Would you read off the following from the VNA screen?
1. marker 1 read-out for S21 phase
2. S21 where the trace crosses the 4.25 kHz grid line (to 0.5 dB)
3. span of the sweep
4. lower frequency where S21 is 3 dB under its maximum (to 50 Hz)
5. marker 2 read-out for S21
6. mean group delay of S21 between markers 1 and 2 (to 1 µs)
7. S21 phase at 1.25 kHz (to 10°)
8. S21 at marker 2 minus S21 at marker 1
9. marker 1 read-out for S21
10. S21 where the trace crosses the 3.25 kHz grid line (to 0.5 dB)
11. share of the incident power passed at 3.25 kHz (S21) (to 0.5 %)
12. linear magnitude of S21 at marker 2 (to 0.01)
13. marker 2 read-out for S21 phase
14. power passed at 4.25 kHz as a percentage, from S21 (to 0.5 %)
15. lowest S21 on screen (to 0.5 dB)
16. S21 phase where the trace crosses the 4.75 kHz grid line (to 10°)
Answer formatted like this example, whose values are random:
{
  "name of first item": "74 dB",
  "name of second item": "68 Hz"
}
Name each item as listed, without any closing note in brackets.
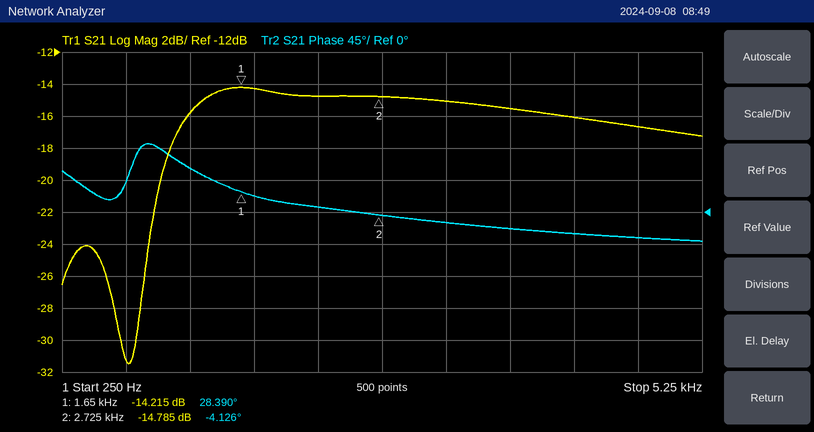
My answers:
{
  "marker 1 read-out for S21 phase": "28.390°",
  "S21 where the trace crosses the 4.25 kHz grid line": "-16.0 dB",
  "span of the sweep": "5 kHz",
  "lower frequency where S21 is 3 dB under its maximum": "1.15 kHz",
  "marker 2 read-out for S21": "-14.785 dB",
  "mean group delay of S21 between markers 1 and 2": "84 µs",
  "S21 phase at 1.25 kHz": "60°",
  "S21 at marker 2 minus S21 at marker 1": "-0.570 dB",
  "marker 1 read-out for S21": "-14.215 dB",
  "S21 where the trace crosses the 3.25 kHz grid line": "-15.0 dB",
  "share of the incident power passed at 3.25 kHz (S21)": "3.0 %",
  "linear magnitude of S21 at marker 2": "0.18",
  "marker 2 read-out for S21 phase": "-4.126°",
  "power passed at 4.25 kHz as a percentage, from S21": "2.5 %",
  "lowest S21 on screen": "-31.5 dB",
  "S21 phase where the trace crosses the 4.75 kHz grid line": "-40°"
}
